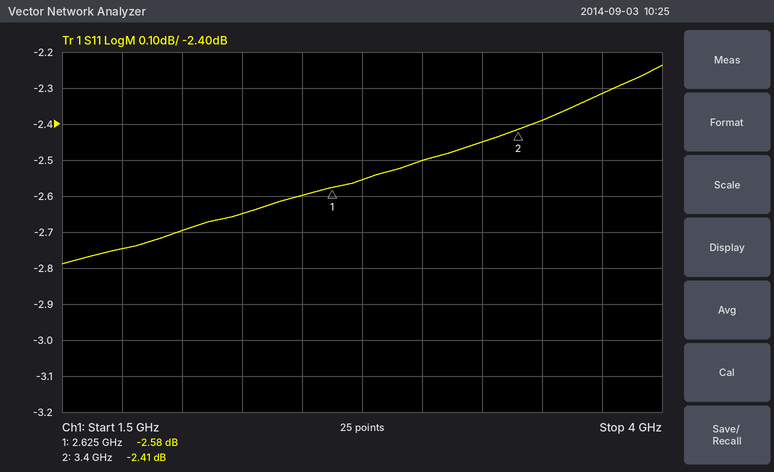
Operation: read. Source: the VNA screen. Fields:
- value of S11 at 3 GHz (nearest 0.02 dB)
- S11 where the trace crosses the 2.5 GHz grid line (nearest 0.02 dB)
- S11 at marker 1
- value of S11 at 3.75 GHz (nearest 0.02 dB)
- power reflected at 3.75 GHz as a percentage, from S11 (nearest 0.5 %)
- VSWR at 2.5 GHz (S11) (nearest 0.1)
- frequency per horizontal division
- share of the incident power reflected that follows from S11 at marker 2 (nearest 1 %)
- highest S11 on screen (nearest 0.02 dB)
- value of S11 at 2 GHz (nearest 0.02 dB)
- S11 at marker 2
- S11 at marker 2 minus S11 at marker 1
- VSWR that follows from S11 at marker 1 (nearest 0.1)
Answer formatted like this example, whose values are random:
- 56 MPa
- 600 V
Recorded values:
- -2.50 dB
- -2.60 dB
- -2.58 dB
- -2.32 dB
- 58.5 %
- 6.7
- 250 MHz
- 57 %
- -2.24 dB
- -2.70 dB
- -2.41 dB
- 0.17 dB
- 6.8
